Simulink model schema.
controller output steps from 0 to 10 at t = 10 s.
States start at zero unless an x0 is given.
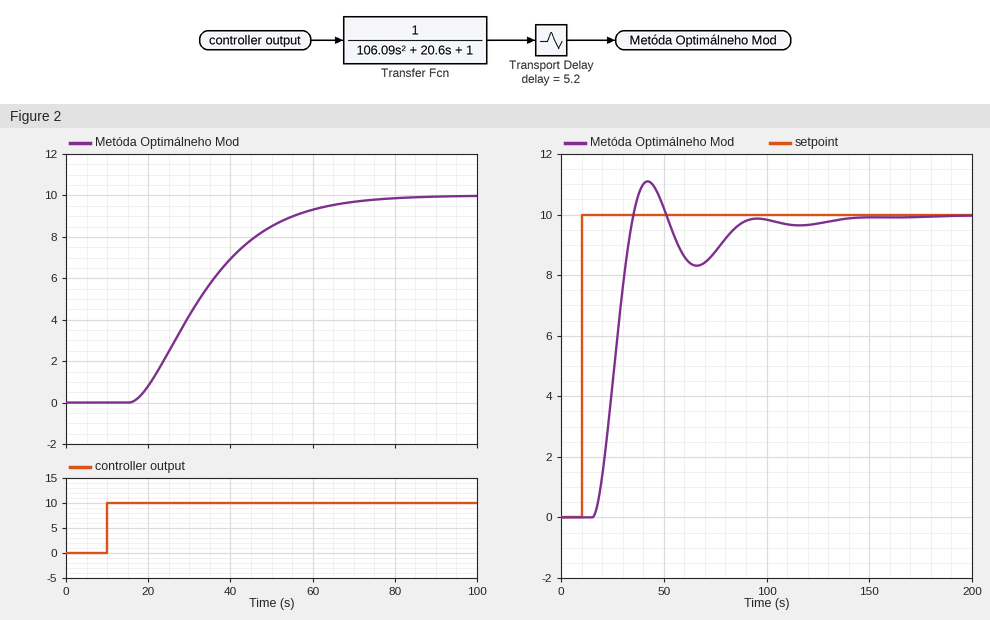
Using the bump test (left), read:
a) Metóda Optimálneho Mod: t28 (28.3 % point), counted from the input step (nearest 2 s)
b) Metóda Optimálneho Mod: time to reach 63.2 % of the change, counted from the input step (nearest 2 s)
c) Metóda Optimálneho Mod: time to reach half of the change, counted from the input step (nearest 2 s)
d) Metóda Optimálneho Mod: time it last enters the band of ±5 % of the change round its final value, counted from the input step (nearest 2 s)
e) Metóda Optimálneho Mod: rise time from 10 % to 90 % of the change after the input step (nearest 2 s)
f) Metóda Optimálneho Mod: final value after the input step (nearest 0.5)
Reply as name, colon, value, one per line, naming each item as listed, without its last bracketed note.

Metóda Optimálneho Mod: t28 (28.3 % point), counted from the input step: 16 s
Metóda Optimálneho Mod: time to reach 63.2 % of the change, counted from the input step: 28 s
Metóda Optimálneho Mod: time to reach half of the change, counted from the input step: 22 s
Metóda Optimálneho Mod: time it last enters the band of ±5 % of the change round its final value, counted from the input step: 54 s
Metóda Optimálneho Mod: rise time from 10 % to 90 % of the change after the input step: 34 s
Metóda Optimálneho Mod: final value after the input step: 10.0
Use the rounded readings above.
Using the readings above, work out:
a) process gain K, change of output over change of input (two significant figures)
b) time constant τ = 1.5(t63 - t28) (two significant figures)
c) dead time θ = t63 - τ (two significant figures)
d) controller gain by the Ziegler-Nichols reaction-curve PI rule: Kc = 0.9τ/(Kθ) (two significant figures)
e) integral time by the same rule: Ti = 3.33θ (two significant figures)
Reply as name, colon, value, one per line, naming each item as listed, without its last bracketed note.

process gain K, change of output over change of input: 1.0
time constant τ = 1.5(t63 - t28): 18 s
dead time θ = t63 - τ: 10 s
controller gain by the Ziegler-Nichols reaction-curve PI rule: Kc = 0.9τ/(Kθ): 1.6
integral time by the same rule: Ti = 3.33θ: 33 s
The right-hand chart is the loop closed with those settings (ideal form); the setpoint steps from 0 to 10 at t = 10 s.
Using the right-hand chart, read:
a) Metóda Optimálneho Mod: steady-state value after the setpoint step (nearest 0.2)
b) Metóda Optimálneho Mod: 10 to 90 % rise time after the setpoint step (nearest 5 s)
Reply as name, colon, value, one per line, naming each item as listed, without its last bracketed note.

Metóda Optimálneho Mod: steady-state value after the setpoint step: 10.0
Metóda Optimálneho Mod: 10 to 90 % rise time after the setpoint step: 15 s
